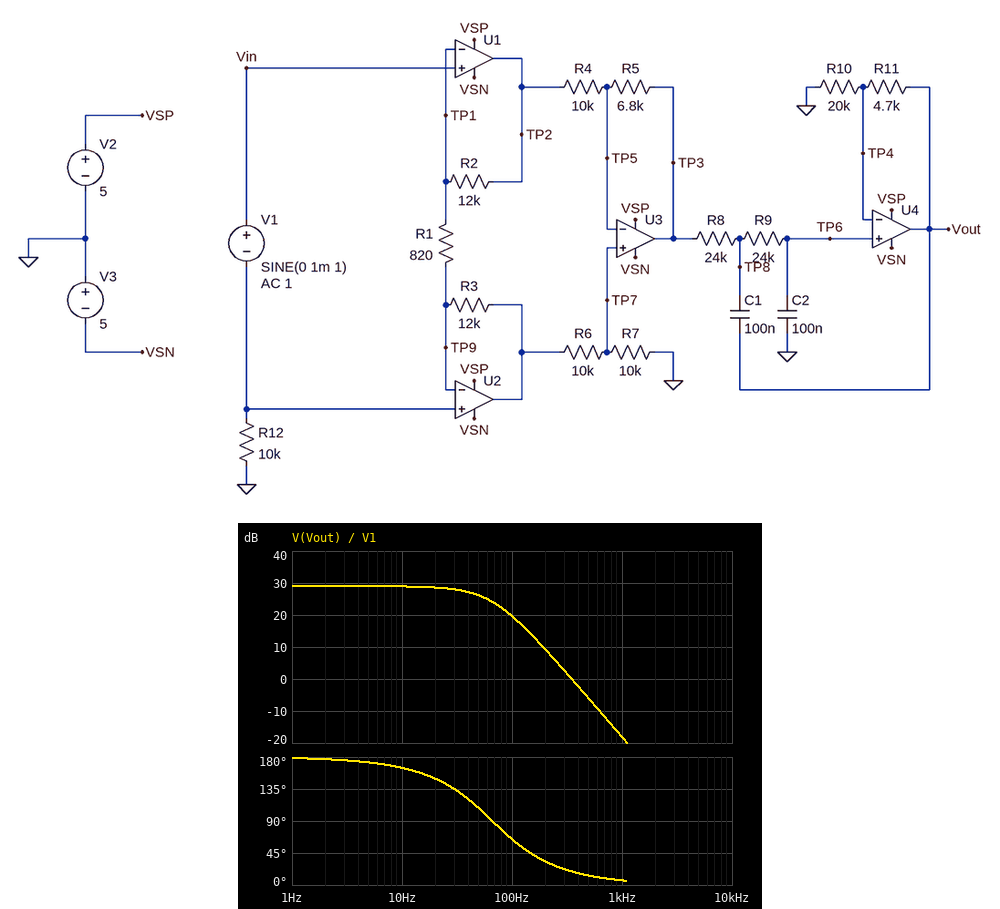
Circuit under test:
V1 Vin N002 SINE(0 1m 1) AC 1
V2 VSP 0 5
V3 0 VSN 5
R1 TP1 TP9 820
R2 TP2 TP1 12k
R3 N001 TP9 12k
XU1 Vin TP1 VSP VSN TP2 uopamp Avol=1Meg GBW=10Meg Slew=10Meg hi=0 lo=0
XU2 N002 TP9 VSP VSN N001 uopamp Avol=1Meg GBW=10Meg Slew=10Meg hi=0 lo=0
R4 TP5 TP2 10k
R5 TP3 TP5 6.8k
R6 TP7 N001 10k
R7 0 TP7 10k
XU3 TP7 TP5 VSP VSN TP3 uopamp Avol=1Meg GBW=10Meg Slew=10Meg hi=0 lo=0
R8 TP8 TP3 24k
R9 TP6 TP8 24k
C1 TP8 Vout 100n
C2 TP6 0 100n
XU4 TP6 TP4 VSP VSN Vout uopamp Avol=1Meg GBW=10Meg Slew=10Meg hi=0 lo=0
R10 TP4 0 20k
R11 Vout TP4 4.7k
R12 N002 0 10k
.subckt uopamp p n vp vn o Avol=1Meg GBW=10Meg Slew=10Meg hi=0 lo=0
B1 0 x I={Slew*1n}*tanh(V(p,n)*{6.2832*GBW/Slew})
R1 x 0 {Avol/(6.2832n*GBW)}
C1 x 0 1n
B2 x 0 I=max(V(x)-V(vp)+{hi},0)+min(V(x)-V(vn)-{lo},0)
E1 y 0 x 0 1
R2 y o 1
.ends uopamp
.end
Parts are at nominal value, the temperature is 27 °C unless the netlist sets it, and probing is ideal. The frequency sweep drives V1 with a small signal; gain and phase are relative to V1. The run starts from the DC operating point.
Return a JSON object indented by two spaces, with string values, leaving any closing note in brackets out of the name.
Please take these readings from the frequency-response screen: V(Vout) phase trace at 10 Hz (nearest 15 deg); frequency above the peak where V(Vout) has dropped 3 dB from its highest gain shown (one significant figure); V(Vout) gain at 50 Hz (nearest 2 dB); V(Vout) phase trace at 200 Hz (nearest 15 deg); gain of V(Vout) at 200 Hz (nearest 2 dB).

{
  "V(Vout) phase trace at 10 Hz": "165 deg",
  "frequency above the peak where V(Vout) has dropped 3 dB from its highest gain shown": "50 Hz",
  "V(Vout) gain at 50 Hz": "26 dB",
  "V(Vout) phase trace at 200 Hz": "30 deg",
  "gain of V(Vout) at 200 Hz": "10 dB"
}
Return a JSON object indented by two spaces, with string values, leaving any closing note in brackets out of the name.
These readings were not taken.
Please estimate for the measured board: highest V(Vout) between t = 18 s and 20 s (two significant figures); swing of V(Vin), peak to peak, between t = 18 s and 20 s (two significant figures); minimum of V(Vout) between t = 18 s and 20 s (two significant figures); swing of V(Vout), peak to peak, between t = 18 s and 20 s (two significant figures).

{
  "highest V(Vout) between t = 18 s and 20 s": "28 mV",
  "swing of V(Vin), peak to peak, between t = 18 s and 20 s": "2.0 mV",
  "minimum of V(Vout) between t = 18 s and 20 s": "-28 mV",
  "swing of V(Vout), peak to peak, between t = 18 s and 20 s": "57 mV"
}
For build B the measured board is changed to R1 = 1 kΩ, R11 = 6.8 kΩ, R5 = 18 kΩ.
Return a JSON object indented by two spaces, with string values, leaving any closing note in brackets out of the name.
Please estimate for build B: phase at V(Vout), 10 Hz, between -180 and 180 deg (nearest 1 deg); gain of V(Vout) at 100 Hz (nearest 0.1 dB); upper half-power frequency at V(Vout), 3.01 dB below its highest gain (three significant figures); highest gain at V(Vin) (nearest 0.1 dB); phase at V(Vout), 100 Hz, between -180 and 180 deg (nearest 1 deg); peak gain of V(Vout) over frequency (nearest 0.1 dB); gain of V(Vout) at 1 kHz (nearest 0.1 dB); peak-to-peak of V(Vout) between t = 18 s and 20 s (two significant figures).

{
  "phase at V(Vout), 10 Hz, between -180 and 180 deg": "166 deg",
  "gain of V(Vout) at 100 Hz": "25.7 dB",
  "upper half-power frequency at V(Vout), 3.01 dB below its highest gain": "55.1 Hz",
  "highest gain at V(Vin)": "0 dB",
  "phase at V(Vout), 100 Hz, between -180 and 180 deg": "63 deg",
  "peak gain of V(Vout) over frequency": "34.6 dB",
  "gain of V(Vout) at 1 kHz": "-12.5 dB",
  "peak-to-peak of V(Vout) between t = 18 s and 20 s": "110 mV"
}
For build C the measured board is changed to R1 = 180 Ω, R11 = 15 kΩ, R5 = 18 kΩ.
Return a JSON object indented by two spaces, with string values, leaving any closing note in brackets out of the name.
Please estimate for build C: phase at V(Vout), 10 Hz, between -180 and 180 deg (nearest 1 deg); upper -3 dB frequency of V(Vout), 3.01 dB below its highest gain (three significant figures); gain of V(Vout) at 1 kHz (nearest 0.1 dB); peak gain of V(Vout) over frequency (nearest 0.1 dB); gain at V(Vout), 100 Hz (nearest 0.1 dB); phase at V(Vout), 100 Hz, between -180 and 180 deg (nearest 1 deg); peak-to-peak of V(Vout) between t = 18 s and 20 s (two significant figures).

{
  "phase at V(Vout), 10 Hz, between -180 and 180 deg": "169 deg",
  "upper -3 dB frequency of V(Vout), 3.01 dB below its highest gain": "72.5 Hz",
  "gain of V(Vout) at 1 kHz": "4.4 dB",
  "peak gain of V(Vout) over frequency": "51.7 dB",
  "gain at V(Vout), 100 Hz": "44.4 dB",
  "phase at V(Vout), 100 Hz, between -180 and 180 deg": "56 deg",
  "peak-to-peak of V(Vout) between t = 18 s and 20 s": "750 mV"
}
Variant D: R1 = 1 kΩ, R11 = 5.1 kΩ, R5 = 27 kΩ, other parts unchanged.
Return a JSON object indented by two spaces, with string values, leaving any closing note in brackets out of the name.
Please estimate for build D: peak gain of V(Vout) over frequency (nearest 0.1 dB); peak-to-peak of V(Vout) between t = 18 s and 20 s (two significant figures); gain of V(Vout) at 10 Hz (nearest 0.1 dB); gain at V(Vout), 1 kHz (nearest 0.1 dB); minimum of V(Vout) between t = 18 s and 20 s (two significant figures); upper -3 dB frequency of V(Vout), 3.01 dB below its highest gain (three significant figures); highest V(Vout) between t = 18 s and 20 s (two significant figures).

{
  "peak gain of V(Vout) over frequency": "37.1 dB",
  "peak-to-peak of V(Vout) between t = 18 s and 20 s": "140 mV",
  "gain of V(Vout) at 10 Hz": "37.0 dB",
  "gain at V(Vout), 1 kHz": "-10.0 dB",
  "minimum of V(Vout) between t = 18 s and 20 s": "-72 mV",
  "upper -3 dB frequency of V(Vout), 3.01 dB below its highest gain": "51.6 Hz",
  "highest V(Vout) between t = 18 s and 20 s": "72 mV"
}
